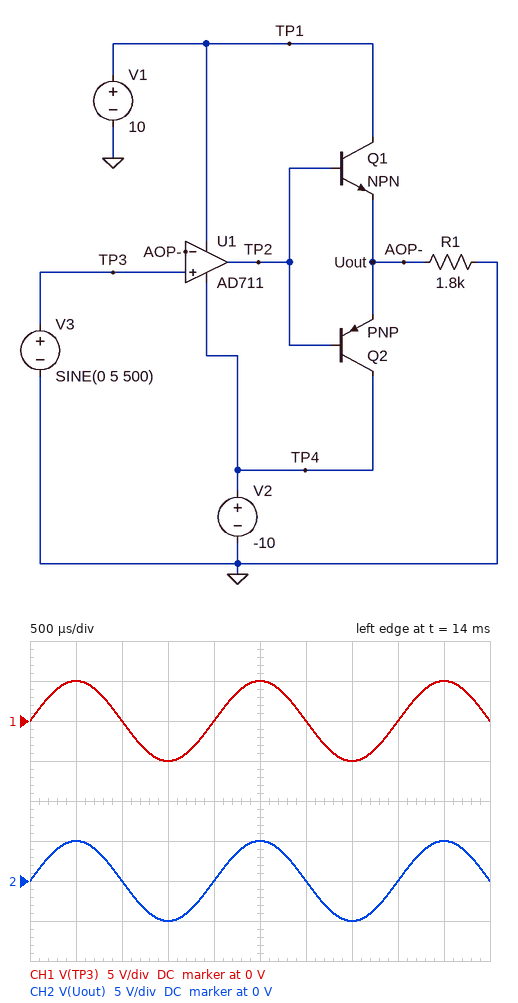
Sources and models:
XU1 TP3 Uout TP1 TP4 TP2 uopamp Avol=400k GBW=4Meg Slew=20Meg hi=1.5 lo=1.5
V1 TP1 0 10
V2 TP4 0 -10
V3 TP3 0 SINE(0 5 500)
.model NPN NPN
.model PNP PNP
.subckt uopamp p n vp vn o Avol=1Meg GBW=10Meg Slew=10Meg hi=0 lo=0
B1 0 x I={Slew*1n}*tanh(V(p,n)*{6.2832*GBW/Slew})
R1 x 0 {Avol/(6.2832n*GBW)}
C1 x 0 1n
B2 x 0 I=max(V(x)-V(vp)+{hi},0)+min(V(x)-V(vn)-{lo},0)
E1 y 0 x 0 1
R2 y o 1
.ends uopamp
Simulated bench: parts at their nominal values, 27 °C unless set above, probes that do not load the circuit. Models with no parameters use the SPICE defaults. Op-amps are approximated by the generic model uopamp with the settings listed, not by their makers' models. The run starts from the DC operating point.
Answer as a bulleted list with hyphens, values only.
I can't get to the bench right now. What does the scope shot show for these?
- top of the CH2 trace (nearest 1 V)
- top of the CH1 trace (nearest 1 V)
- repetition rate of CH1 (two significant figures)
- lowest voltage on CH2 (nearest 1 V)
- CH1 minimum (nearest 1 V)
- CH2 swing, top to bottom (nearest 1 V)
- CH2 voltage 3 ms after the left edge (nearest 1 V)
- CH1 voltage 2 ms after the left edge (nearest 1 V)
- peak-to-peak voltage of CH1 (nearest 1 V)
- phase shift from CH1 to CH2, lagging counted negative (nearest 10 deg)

- 5 V
- 5 V
- 500 Hz
- -5 V
- -5 V
- 10 V
- 0 V
- 0 V
- 10 V
- 0 deg
